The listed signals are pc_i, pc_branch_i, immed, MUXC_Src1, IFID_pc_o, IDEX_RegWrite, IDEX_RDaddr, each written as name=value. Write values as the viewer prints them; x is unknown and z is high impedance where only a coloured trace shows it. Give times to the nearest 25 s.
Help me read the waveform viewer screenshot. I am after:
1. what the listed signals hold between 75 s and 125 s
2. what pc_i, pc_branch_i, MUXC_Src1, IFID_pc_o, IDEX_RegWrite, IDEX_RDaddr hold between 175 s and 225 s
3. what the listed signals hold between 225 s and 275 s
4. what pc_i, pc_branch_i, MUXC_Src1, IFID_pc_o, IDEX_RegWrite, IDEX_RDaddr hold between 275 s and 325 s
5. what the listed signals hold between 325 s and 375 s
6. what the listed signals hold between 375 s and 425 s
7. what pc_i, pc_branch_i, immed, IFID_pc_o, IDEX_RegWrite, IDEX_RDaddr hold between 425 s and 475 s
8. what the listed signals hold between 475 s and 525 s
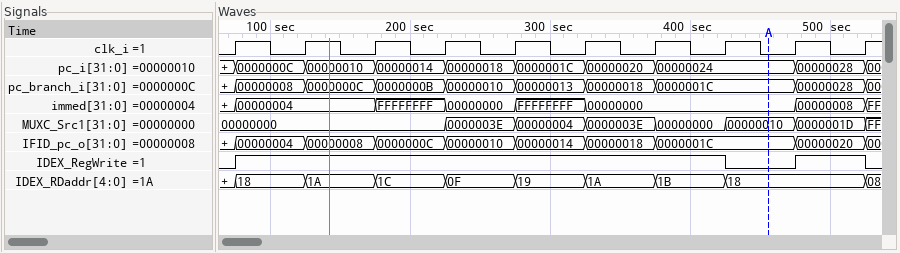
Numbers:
pc_i=0000000C, pc_branch_i=00000008, immed=00000004, MUXC_Src1=00000000, IFID_pc_o=00000004, IDEX_RegWrite=1, IDEX_RDaddr=18
pc_i=00000014, pc_branch_i=0000000B, MUXC_Src1=00000000, IFID_pc_o=0000000C, IDEX_RegWrite=1, IDEX_RDaddr=1C
pc_i=00000018, pc_branch_i=00000010, immed=00000000, MUXC_Src1=0000003E, IFID_pc_o=00000010, IDEX_RegWrite=1, IDEX_RDaddr=0F
pc_i=0000001C, pc_branch_i=00000013, MUXC_Src1=00000004, IFID_pc_o=00000014, IDEX_RegWrite=1, IDEX_RDaddr=19
pc_i=00000020, pc_branch_i=00000018, immed=00000000, MUXC_Src1=0000003E, IFID_pc_o=00000018, IDEX_RegWrite=1, IDEX_RDaddr=1A
pc_i=00000024, pc_branch_i=0000001C, immed=00000000, MUXC_Src1=00000000, IFID_pc_o=0000001C, IDEX_RegWrite=1, IDEX_RDaddr=1B
pc_i=00000024, pc_branch_i=0000001C, immed=00000000, IFID_pc_o=0000001C, IDEX_RegWrite=0, IDEX_RDaddr=18
pc_i=00000028, pc_branch_i=00000028, immed=00000008, MUXC_Src1=0000001D, IFID_pc_o=00000020, IDEX_RegWrite=1, IDEX_RDaddr=18
